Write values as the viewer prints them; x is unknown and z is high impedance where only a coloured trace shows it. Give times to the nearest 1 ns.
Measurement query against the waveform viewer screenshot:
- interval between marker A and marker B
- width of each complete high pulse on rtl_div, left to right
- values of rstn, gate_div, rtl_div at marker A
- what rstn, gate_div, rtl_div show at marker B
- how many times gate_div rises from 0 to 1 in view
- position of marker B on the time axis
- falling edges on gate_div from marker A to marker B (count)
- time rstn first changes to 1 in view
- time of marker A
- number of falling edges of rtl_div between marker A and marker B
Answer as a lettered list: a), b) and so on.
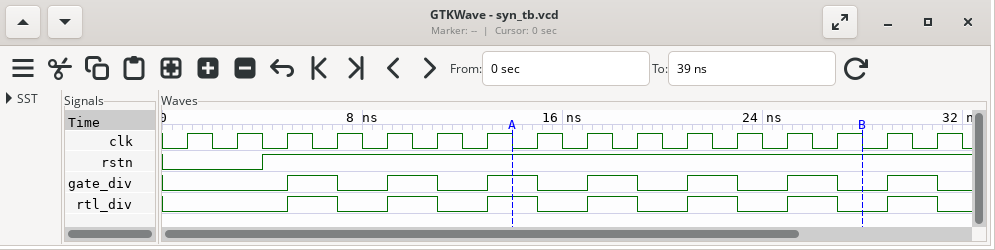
a) 14 ns
b) 2 ns, 2 ns, 2 ns, 2 ns, 2 ns, 2 ns, 2 ns
c) rstn=1, gate_div=1, rtl_div=1
d) rstn=1, gate_div=0, rtl_div=0
e) 7
f) 28 ns
g) 4
h) 4 ns
i) 14 ns
j) 4
